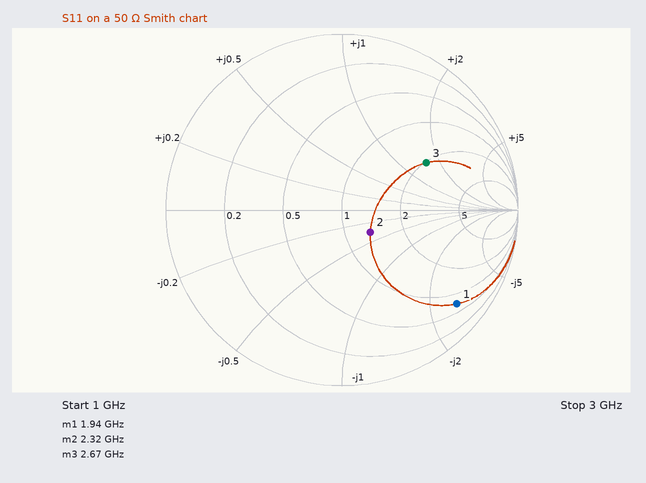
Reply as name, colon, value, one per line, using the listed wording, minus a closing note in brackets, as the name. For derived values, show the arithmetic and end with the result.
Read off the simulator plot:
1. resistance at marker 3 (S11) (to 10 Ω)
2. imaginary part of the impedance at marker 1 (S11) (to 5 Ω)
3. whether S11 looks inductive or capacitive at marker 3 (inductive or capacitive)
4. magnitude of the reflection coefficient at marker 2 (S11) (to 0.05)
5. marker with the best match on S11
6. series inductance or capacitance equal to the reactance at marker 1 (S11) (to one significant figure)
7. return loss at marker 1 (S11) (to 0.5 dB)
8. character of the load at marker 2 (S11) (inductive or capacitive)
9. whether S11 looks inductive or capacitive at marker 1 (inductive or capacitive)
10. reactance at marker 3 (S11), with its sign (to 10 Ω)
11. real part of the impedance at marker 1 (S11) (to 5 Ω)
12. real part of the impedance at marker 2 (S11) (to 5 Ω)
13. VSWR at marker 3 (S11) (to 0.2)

resistance at marker 3 (S11): 100 Ω
imaginary part of the impedance at marker 1 (S11): -130 Ω
whether S11 looks inductive or capacitive at marker 3: inductive
magnitude of the reflection coefficient at marker 2 (S11): 0.20
marker with the best match on S11: marker 2
series inductance or capacitance equal to the reactance at marker 1 (S11): C = 1/(2π × 1.94 GHz × 130 Ω) ≈ 631 fF, so 600 fF to one significant figure
return loss at marker 1 (S11): 1.5 dB
character of the load at marker 2 (S11): capacitive
whether S11 looks inductive or capacitive at marker 1: capacitive
reactance at marker 3 (S11), with its sign: +80 Ω
real part of the impedance at marker 1 (S11): 35 Ω
real part of the impedance at marker 2 (S11): 65 Ω
VSWR at marker 3 (S11): 3.4
